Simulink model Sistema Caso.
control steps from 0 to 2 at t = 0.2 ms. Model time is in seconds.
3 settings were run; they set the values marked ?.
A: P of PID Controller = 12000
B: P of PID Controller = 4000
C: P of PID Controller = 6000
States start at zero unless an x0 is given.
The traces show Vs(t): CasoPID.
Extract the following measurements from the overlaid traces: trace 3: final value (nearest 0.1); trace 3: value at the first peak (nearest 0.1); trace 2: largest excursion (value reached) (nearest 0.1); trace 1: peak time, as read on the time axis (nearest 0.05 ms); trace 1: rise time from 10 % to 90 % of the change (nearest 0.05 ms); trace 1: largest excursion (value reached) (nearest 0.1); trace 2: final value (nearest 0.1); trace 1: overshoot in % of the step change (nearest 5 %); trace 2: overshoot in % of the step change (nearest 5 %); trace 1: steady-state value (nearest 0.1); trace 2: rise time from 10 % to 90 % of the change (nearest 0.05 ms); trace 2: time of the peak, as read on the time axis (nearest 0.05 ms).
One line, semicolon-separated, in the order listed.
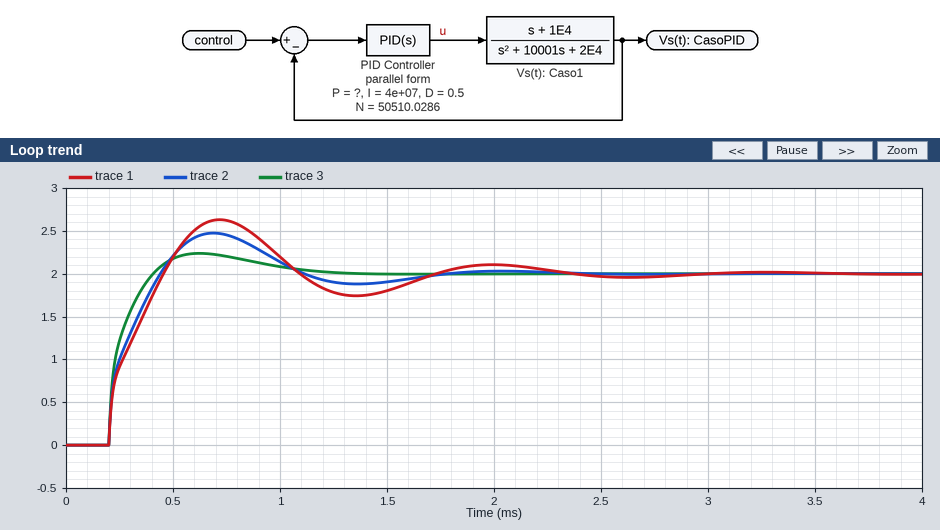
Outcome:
2.0; 2.2; 2.5; 0.70 ms; 0.20 ms; 2.6; 2.0; 30 %; 25 %; 2.0; 0.20 ms; 0.70 ms
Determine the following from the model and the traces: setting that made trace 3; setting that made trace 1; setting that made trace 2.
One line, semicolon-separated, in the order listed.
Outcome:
A; B; C
